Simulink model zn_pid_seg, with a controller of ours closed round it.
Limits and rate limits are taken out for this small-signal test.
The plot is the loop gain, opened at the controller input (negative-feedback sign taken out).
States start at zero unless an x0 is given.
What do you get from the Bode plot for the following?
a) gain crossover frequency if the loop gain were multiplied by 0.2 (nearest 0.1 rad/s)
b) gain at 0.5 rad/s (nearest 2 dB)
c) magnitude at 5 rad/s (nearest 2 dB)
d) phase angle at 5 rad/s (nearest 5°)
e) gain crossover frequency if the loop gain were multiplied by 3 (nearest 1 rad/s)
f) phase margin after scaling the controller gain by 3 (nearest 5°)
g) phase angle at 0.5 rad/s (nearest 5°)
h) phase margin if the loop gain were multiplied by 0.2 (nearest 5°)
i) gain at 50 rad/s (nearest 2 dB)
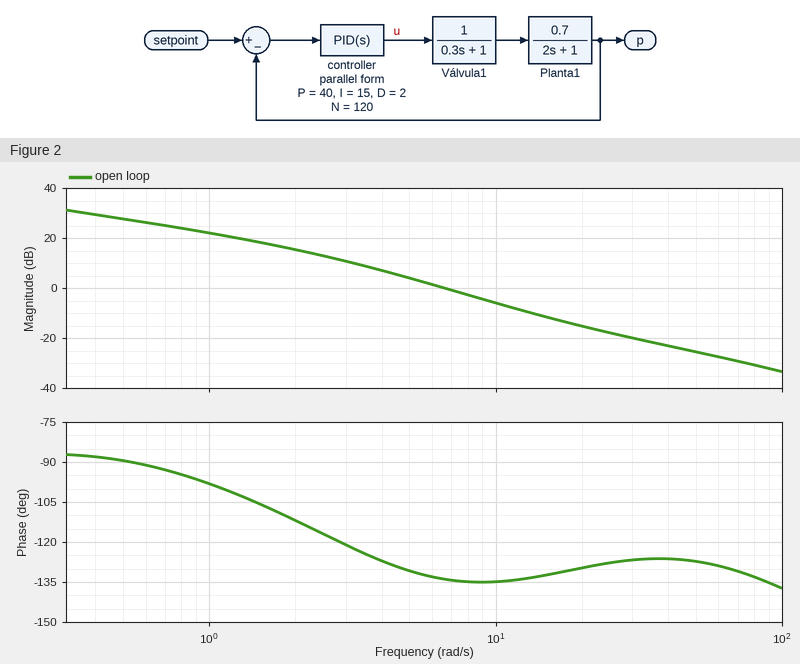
2.3 rad/s
28 dB
4 dB
-130°
13 rad/s
45°
-90°
65°
-26 dB
